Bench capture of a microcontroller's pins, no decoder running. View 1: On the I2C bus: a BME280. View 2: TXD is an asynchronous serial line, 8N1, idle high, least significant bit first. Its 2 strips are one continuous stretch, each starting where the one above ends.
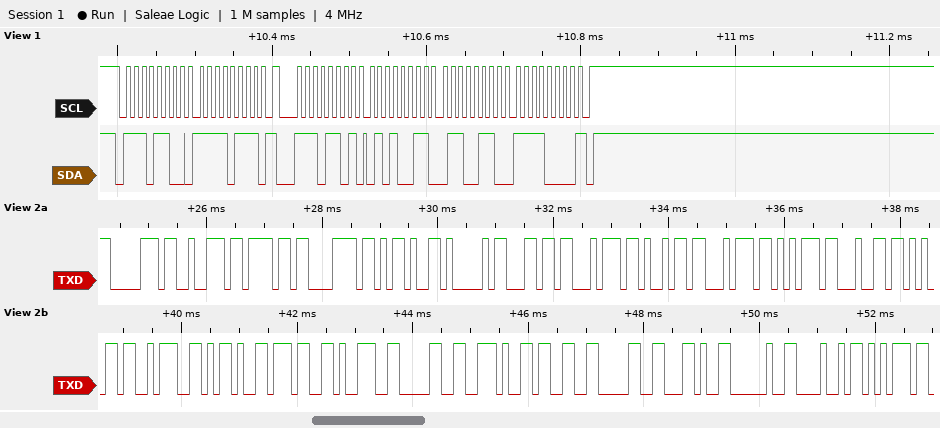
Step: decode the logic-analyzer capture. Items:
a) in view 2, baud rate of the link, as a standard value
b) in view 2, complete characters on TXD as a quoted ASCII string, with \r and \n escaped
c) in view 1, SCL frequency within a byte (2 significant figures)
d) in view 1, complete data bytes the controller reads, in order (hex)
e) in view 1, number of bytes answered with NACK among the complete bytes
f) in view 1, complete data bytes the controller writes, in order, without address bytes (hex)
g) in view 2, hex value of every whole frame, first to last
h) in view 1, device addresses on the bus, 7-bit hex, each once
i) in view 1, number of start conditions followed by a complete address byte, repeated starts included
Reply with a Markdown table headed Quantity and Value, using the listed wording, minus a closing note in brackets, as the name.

| Quantity | Value |
|---|---|
| in view 2, baud rate of the link, as a standard value | 9600 baud |
| in view 2, complete characters on TXD as a quoted ASCII string, with \r and \n escaped | "prox-Altitude:-790.30, Hu" |
| in view 1, SCL frequency within a byte | 100 kHz |
| in view 1, complete data bytes the controller reads, in order | 53 66 F0 |
| in view 1, number of bytes answered with NACK among the complete bytes | 1 |
| in view 1, complete data bytes the controller writes, in order, without address bytes | F7 |
| in view 2, hex value of every whole frame, first to last | 70 72 6F 78 2D 41 6C 74 69 74 75 64 65 3A 2D 37 39 30 2E 33 30 2C 20 48 75 |
| in view 1, device addresses on the bus, 7-bit hex, each once | 0x76 |
| in view 1, number of start conditions followed by a complete address byte, repeated starts included | 2 |
